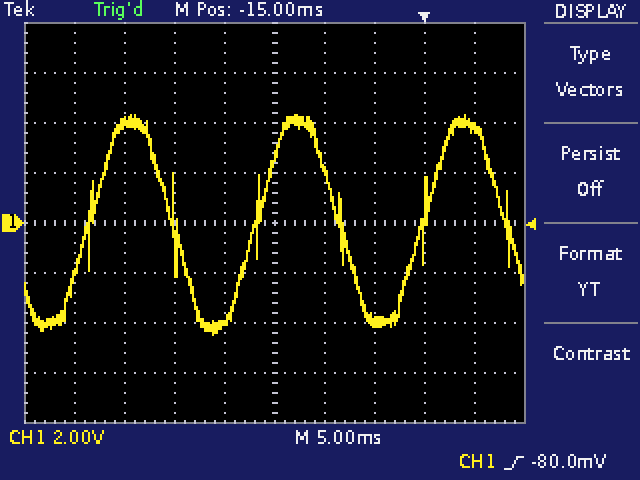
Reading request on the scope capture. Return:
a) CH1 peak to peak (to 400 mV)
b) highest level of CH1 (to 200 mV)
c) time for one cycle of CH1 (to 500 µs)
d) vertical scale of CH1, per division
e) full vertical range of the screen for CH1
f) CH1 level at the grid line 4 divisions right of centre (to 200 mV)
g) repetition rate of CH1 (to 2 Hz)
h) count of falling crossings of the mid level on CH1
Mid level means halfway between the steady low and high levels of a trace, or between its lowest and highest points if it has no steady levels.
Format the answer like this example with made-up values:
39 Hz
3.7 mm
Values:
8.8 V
4.4 V
16.5 ms
2 V
16 V
3.8 V
60 Hz
3
